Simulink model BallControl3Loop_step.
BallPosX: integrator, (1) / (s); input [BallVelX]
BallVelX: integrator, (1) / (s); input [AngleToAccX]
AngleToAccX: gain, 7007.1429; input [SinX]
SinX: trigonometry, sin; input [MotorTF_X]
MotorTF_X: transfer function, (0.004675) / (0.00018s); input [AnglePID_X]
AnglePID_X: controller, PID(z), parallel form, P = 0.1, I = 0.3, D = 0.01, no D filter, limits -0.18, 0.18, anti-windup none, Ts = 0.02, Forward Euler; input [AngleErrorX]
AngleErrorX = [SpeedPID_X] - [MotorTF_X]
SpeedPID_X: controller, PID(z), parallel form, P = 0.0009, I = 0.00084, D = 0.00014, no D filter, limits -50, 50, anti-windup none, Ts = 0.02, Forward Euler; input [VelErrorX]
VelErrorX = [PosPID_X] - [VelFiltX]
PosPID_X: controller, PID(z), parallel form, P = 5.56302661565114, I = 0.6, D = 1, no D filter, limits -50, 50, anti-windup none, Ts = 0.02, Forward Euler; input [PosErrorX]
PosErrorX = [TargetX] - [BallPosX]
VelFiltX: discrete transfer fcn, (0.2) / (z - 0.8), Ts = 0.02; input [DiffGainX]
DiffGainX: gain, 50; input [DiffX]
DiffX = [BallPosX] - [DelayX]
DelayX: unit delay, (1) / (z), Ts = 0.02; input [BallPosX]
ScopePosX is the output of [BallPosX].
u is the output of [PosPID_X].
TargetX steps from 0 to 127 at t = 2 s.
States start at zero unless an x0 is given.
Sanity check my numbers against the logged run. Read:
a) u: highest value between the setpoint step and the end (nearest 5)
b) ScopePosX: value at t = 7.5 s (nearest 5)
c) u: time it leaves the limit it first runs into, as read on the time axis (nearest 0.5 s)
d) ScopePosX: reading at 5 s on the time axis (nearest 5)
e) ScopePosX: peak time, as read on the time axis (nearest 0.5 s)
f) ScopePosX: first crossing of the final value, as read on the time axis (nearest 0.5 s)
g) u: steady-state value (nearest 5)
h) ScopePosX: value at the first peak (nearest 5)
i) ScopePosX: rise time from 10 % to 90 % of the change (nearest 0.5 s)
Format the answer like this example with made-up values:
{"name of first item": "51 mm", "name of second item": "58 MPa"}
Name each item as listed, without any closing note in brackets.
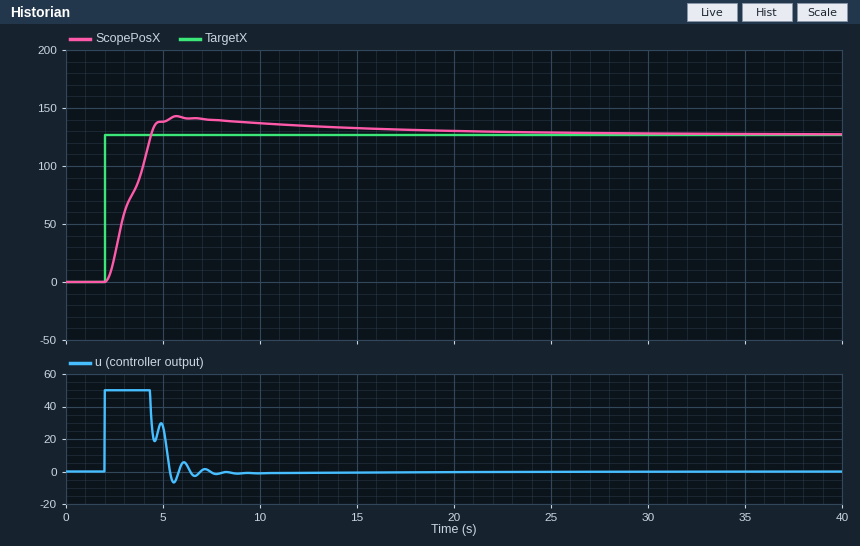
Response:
{"u: highest value between the setpoint step and the end": "50", "ScopePosX: value at t = 7.5 s": "140", "u: time it leaves the limit it first runs into, as read on the time axis": "4.5 s", "ScopePosX: reading at 5 s on the time axis": "140", "ScopePosX: peak time, as read on the time axis": "5.5 s", "ScopePosX: first crossing of the final value, as read on the time axis": "4.5 s", "u: steady-state value": "0", "ScopePosX: value at the first peak": "145", "ScopePosX: rise time from 10 % to 90 % of the change": "2.0 s"}
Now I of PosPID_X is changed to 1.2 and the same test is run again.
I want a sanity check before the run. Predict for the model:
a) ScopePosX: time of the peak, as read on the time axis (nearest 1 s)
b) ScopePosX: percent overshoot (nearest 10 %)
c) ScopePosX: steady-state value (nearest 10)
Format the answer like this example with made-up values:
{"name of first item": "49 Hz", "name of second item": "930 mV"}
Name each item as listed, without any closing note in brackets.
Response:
{"ScopePosX: time of the peak, as read on the time axis": "6 s", "ScopePosX: percent overshoot": "20 %", "ScopePosX: steady-state value": "130"}
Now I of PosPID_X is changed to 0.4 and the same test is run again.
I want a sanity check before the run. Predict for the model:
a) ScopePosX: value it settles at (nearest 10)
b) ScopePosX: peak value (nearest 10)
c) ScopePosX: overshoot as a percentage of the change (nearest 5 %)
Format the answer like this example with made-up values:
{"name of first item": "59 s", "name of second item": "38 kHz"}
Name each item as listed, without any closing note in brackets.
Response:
{"ScopePosX: value it settles at": "130", "ScopePosX: peak value": "140", "ScopePosX: overshoot as a percentage of the change": "10 %"}
